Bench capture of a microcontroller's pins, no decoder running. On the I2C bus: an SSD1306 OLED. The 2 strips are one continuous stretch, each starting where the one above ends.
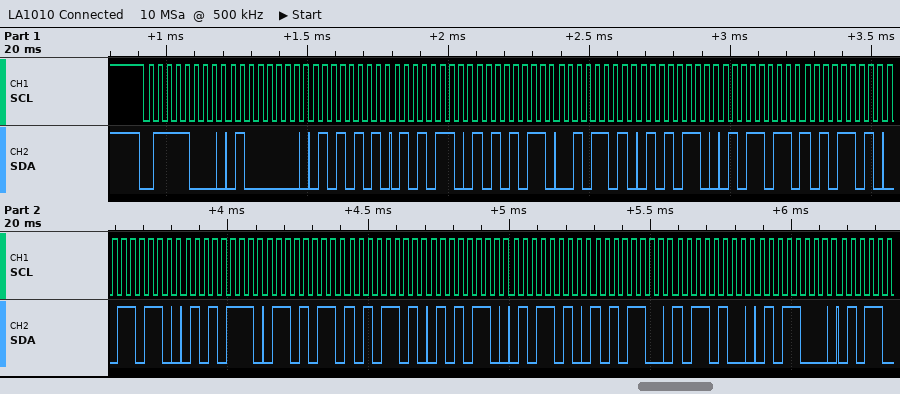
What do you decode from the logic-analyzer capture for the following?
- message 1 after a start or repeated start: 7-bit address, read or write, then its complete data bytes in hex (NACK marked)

0x3C write: 40 55 56 AB 2D 56 5B AD 36 57 6B AD 56 5A AC B4 58
